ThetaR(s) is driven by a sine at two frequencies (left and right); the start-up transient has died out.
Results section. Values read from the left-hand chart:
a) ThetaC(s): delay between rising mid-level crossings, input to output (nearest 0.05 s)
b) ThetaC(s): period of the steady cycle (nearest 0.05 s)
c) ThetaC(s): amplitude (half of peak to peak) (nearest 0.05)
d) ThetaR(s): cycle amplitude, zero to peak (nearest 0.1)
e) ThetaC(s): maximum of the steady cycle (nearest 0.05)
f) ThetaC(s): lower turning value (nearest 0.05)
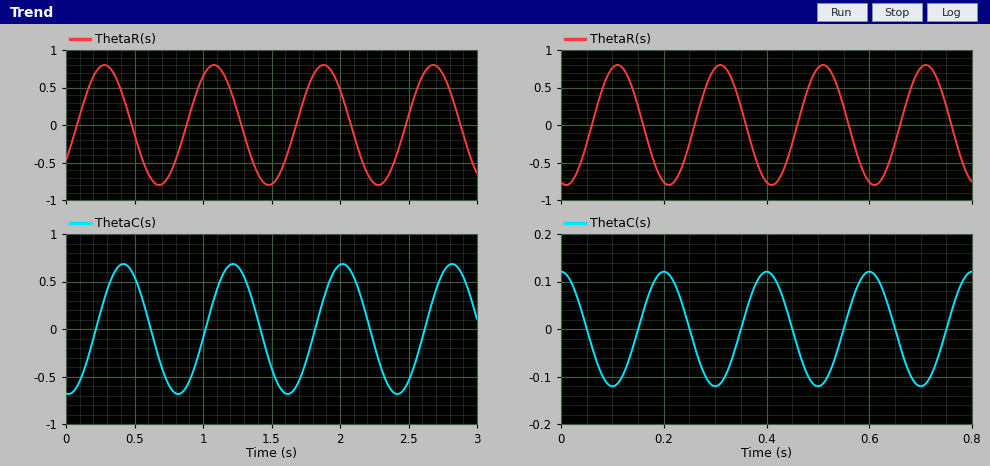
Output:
0.15 s
0.80 s
0.70
0.8
0.70
-0.70
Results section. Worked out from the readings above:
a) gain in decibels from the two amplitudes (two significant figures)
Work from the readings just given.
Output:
-1.2 dB
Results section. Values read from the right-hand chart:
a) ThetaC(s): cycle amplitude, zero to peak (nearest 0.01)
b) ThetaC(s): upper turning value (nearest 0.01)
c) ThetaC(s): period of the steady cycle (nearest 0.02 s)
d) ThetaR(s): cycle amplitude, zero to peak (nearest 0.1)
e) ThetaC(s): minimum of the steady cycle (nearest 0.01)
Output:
0.12
0.12
0.20 s
0.8
-0.12
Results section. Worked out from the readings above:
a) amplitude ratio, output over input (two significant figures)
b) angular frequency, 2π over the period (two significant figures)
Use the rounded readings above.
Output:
0.15
31 rad/s
